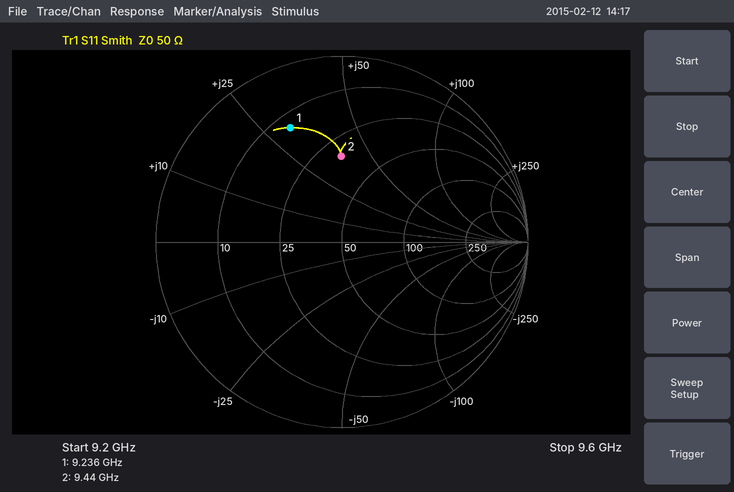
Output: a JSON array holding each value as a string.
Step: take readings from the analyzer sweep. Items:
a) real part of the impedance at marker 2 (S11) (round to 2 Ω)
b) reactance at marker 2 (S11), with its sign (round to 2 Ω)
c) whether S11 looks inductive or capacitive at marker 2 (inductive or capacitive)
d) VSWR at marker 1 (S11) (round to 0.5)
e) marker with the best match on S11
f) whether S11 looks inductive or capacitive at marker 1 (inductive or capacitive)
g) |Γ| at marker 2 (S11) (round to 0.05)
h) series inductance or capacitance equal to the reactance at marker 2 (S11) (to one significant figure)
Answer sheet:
["32 Ω", "+38 Ω", "inductive", "5.0", "marker 2", "inductive", "0.45", "600 pH"]
